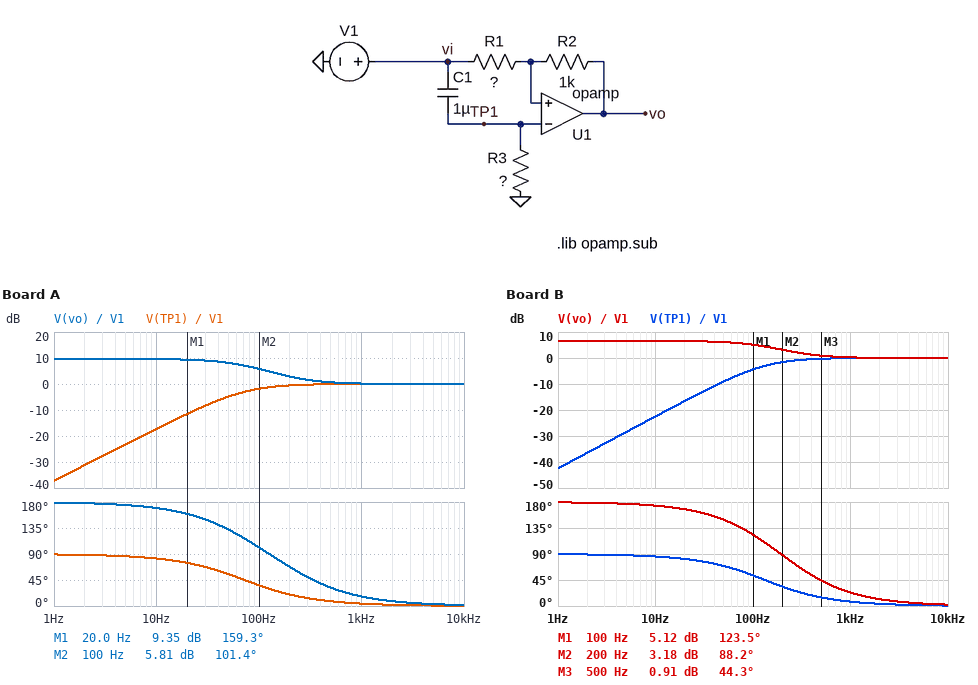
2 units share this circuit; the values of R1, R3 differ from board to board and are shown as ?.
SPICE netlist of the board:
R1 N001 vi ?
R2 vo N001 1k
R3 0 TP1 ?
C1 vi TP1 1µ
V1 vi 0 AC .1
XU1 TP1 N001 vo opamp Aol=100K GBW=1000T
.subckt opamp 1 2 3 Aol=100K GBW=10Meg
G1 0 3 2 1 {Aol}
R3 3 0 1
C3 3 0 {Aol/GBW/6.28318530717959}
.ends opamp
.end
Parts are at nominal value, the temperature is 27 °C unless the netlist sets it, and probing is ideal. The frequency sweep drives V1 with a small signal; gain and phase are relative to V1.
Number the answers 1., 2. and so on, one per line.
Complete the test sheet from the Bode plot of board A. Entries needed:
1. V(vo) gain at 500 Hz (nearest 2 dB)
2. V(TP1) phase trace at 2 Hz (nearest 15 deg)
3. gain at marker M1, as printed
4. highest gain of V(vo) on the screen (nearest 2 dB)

1. 0 dB
2. 90 deg
3. 9.35 dB
4. 10 dB
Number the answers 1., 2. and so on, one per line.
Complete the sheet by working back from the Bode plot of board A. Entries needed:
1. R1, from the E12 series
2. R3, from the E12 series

1. 330 Ω
2. 2.2 kΩ
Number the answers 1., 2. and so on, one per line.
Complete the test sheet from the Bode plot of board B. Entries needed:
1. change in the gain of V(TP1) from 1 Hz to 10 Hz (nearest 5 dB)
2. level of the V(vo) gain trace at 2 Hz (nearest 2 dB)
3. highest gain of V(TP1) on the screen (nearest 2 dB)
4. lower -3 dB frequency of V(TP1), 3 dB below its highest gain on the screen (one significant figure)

1. 20 dB
2. 6 dB
3. 0 dB
4. 100 Hz
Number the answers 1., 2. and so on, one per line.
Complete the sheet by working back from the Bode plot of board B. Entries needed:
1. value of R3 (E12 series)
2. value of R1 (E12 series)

1. 1.2 kΩ
2. 470 Ω
